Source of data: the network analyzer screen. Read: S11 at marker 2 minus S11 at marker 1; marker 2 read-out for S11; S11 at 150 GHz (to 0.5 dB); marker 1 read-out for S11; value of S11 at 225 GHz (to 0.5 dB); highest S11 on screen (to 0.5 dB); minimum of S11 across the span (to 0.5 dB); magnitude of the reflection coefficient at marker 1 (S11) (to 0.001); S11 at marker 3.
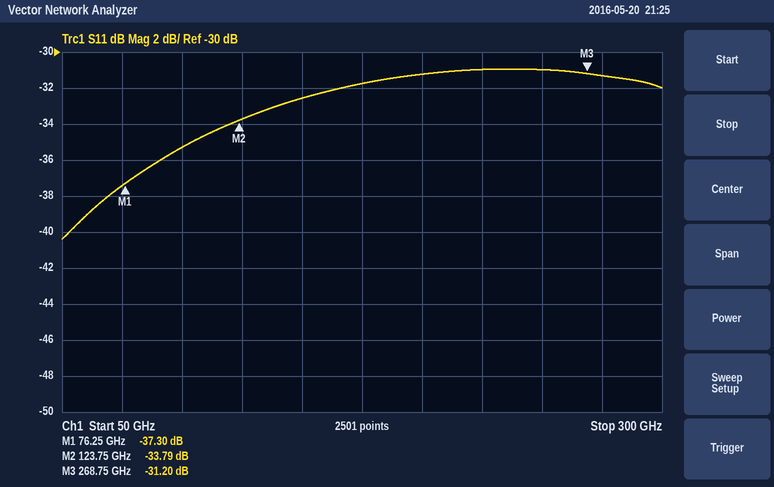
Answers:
3.51 dB
-33.79 dB
-32.5 dB
-37.30 dB
-31.0 dB
-31.0 dB
-40.5 dB
0.014
-31.20 dB
